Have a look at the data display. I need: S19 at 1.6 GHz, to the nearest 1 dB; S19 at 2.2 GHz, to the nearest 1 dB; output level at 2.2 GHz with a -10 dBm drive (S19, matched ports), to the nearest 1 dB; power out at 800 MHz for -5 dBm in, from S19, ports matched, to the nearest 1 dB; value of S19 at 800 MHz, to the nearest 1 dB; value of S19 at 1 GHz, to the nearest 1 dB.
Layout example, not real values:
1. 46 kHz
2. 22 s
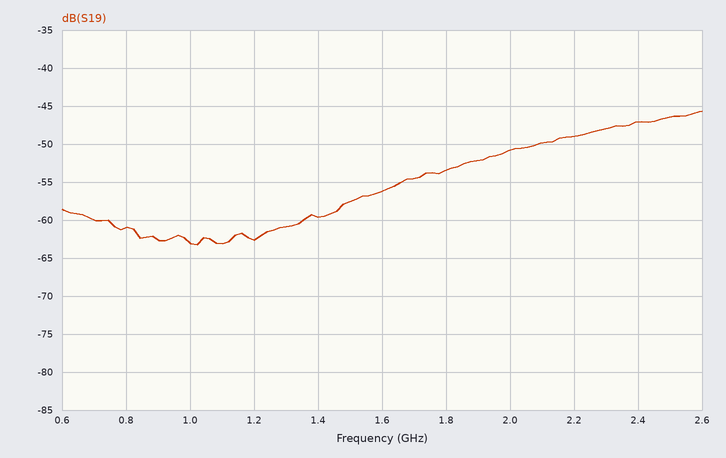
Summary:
1. -56 dB
2. -49 dB
3. -59 dBm
4. -66 dBm
5. -61 dB
6. -63 dB
